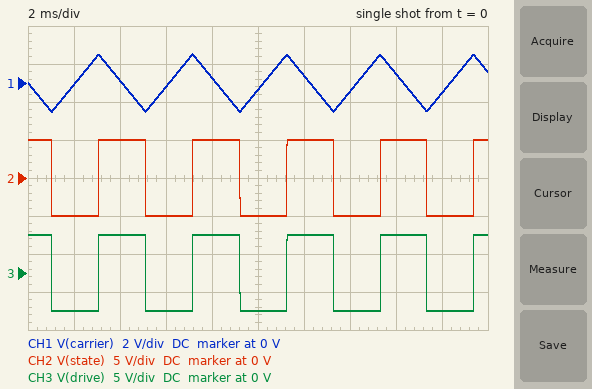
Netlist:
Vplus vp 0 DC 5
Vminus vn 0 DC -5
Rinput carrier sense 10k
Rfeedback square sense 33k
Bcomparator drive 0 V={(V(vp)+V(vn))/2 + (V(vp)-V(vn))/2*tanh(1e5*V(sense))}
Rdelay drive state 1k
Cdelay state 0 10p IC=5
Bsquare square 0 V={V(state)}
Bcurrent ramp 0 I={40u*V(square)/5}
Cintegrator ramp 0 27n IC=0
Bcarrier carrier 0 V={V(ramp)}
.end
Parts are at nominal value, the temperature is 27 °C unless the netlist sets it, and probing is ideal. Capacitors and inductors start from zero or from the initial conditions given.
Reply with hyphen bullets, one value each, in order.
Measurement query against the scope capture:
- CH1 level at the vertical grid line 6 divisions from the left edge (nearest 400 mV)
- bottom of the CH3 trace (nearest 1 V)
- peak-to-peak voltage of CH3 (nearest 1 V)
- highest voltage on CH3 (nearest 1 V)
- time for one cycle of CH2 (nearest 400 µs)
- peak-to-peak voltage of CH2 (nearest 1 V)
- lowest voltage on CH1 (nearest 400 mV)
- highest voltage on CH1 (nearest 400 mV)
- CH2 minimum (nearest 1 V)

- 400 mV
- -5 V
- 10 V
- 5 V
- 4.0 ms
- 10 V
- -1.6 V
- 1.6 V
- -5 V
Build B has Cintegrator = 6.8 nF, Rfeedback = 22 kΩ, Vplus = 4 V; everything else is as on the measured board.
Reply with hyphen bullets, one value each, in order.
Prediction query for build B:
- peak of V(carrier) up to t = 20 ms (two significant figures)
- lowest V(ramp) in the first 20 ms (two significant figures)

- 2.3 V
- -1.8 V
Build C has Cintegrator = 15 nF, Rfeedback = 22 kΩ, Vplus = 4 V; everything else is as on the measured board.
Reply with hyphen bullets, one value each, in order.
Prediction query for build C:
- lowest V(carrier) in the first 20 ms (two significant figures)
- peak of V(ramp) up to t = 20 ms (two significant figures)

- -1.8 V
- 2.3 V
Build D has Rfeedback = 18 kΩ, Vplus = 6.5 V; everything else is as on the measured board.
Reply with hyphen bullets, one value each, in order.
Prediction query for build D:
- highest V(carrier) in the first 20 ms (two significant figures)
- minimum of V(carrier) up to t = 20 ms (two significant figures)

- 2.8 V
- -3.6 V
